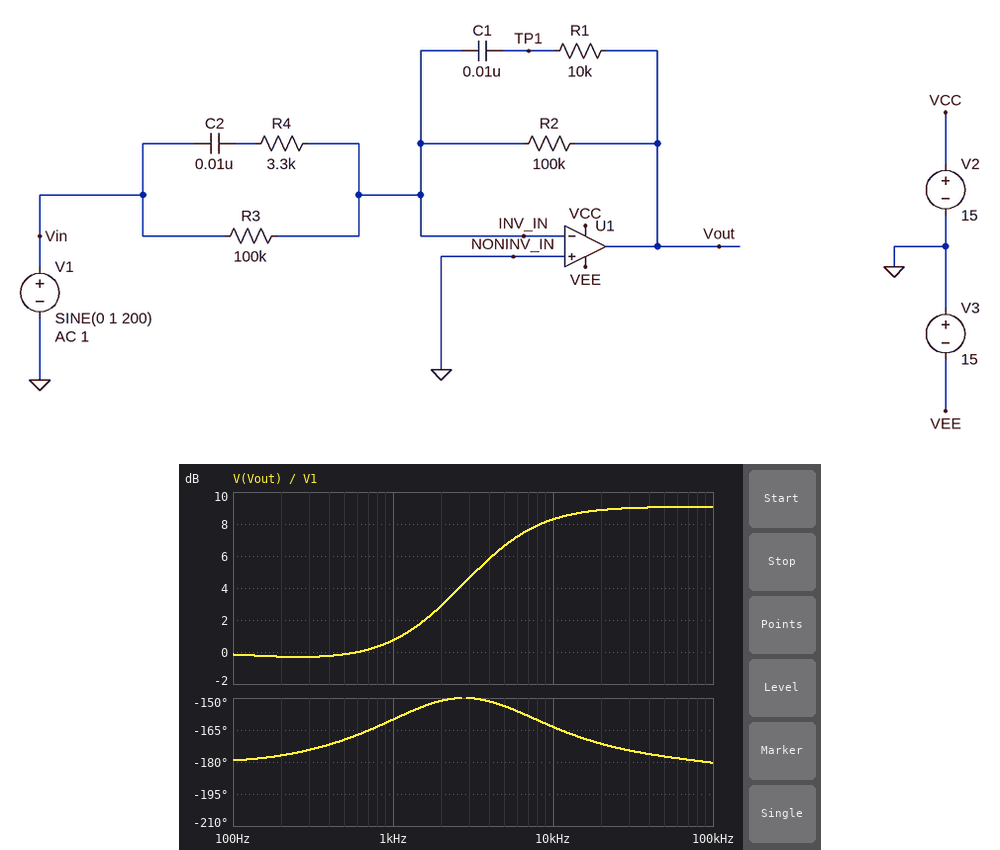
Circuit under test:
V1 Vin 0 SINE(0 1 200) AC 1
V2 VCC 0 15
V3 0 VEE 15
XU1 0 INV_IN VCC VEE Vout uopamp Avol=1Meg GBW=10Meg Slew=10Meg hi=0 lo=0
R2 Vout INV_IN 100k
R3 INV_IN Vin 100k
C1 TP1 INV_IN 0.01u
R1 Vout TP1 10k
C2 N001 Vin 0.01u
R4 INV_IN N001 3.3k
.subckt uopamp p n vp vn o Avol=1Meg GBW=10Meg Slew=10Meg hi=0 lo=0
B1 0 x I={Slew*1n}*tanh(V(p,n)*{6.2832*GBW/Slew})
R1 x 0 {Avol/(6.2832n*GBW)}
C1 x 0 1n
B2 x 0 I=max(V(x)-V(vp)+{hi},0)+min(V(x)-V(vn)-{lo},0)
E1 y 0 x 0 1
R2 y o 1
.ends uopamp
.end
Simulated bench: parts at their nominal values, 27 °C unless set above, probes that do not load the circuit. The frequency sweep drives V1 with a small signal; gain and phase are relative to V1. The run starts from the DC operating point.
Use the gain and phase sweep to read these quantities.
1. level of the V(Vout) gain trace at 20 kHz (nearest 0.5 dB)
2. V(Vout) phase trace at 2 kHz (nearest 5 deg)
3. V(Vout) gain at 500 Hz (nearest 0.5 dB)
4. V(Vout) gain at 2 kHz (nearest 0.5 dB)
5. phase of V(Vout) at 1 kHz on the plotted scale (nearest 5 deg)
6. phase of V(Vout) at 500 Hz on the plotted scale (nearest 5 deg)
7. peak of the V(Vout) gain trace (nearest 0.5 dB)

9.0 dB
-150 deg
0 dB
3.0 dB
-160 deg
-170 deg
9.0 dB
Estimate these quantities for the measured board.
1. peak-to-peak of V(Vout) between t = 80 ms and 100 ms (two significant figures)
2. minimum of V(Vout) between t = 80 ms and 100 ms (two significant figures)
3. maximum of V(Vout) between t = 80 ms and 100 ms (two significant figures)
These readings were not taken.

1.9 V
-970 mV
970 mV
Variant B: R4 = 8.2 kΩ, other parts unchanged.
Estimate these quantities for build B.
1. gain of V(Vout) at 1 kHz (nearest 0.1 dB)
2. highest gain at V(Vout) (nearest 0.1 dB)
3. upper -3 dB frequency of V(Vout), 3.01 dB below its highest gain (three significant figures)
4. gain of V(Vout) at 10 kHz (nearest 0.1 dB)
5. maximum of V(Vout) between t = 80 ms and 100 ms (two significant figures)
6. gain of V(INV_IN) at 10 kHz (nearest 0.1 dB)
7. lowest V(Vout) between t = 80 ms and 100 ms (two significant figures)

0.3 dB
1.6 dB
4.55 MHz
1.5 dB
990 mV
-58.5 dB
-990 mV
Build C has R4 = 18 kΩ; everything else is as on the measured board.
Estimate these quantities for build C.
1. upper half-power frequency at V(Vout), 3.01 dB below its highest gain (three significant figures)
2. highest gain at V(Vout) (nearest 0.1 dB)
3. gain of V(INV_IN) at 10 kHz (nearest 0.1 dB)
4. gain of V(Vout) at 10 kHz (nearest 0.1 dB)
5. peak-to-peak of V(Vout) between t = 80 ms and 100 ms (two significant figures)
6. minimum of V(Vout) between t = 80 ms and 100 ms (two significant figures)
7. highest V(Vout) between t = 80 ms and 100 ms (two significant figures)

1.66 kHz
0.3 dB
-64.4 dB
-4.4 dB
2.1 V
-1.0 V
1.0 V
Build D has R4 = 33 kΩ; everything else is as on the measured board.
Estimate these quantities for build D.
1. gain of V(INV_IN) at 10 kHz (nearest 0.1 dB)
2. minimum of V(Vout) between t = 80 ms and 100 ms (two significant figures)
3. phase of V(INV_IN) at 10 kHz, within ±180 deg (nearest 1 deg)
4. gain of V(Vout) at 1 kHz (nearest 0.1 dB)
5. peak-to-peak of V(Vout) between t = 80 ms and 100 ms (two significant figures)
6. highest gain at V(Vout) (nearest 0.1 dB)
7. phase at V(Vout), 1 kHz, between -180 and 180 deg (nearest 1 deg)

-68.6 dB
-1.1 V
84 deg
-4.2 dB
2.1 V
0.6 dB
149 deg
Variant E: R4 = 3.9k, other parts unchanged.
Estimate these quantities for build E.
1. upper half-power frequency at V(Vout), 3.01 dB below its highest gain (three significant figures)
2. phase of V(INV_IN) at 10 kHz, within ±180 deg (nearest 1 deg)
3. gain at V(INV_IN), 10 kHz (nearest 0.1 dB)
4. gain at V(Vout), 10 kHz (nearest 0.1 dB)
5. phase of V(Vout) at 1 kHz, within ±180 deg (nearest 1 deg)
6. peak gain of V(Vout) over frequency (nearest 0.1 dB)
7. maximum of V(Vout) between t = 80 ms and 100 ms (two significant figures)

2.93 MHz
103 deg
-52.9 dB
7.1 dB
-162 deg
7.7 dB
970 mV
